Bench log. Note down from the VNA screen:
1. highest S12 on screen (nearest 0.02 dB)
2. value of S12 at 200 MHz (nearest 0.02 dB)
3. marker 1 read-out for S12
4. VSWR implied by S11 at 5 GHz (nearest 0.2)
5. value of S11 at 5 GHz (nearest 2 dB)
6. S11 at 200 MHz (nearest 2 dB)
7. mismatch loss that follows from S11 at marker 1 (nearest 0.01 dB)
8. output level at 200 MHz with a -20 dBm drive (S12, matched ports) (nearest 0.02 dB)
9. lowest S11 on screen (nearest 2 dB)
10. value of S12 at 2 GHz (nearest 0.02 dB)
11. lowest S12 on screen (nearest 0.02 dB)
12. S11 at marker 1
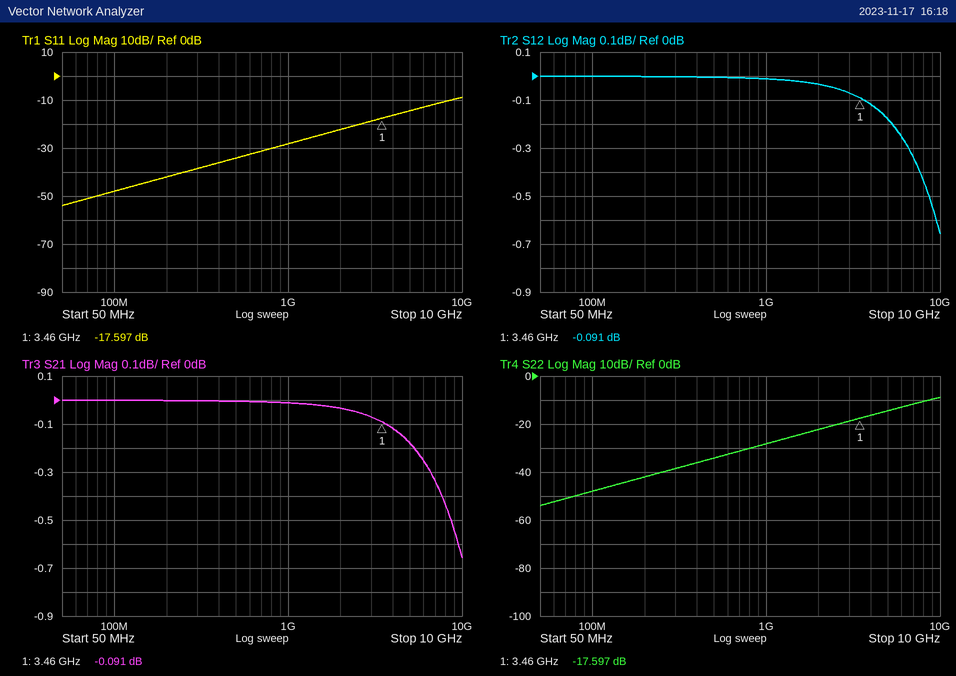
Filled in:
0.00 dB
0.00 dB
-0.091 dB
1.4
-14 dB
-42 dB
0.08 dB
-20.00 dBm
-54 dB
-0.04 dB
-0.66 dB
-17.597 dB
